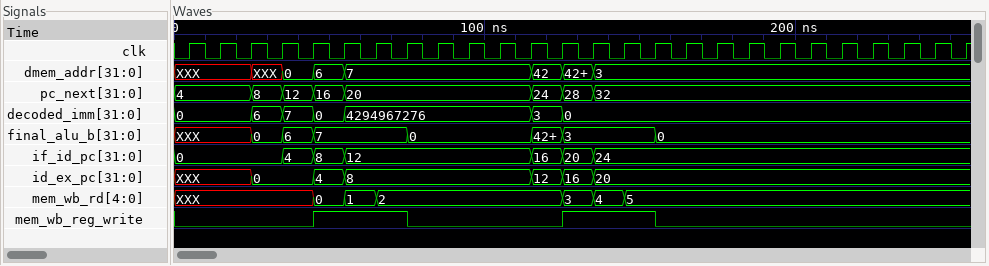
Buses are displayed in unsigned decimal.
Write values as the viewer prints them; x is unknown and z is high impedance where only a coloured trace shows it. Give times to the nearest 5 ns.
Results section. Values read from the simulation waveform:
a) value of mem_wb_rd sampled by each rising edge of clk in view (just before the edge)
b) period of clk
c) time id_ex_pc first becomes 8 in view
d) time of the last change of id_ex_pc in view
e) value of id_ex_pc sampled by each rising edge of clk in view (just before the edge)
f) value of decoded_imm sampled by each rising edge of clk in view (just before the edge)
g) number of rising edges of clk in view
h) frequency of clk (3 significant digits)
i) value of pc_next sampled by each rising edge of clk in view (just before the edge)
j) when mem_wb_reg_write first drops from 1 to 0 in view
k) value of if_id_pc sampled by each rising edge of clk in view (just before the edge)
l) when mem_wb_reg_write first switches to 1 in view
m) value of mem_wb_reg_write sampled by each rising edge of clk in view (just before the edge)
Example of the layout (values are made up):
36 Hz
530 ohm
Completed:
XXX, XXX, XXX, XXX, XXX, 0, 1, 2, 2, 2, 2, 2, 2, 3, 4, 5, 5, 5, 5, 5, 5, 5, 5, 5, 5, 5
10 ns
55 ns
135 ns
XXX, XXX, XXX, 0, 0, 4, 8, 8, 8, 8, 8, 8, 12, 16, 20, 20, 20, 20, 20, 20, 20, 20, 20, 20, 20, 20
0, 0, 0, 6, 7, 0, 4294967276, 4294967276, 4294967276, 4294967276, 4294967276, 4294967276, 3, 0, 0, 0, 0, 0, 0, 0, 0, 0, 0, 0, 0, 0
26
100 MHz
4, 4, 4, 8, 12, 16, 20, 20, 20, 20, 20, 20, 24, 28, 32, 32, 32, 32, 32, 32, 32, 32, 32, 32, 32, 32
75 ns
0, 0, 0, 0, 4, 8, 12, 12, 12, 12, 12, 12, 16, 20, 24, 24, 24, 24, 24, 24, 24, 24, 24, 24, 24, 24
45 ns
0 0 0 0 0 1 1 1 0 0 0 0 0 1 1 1 0 0 0 0 0 0 0 0 0 0
